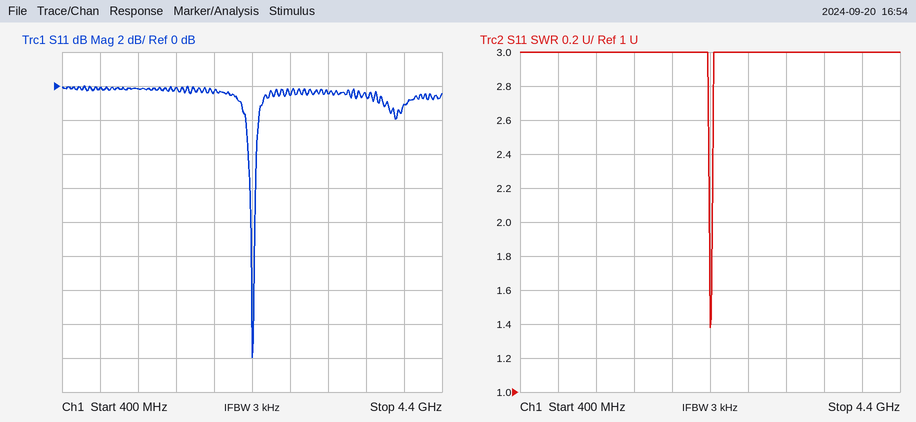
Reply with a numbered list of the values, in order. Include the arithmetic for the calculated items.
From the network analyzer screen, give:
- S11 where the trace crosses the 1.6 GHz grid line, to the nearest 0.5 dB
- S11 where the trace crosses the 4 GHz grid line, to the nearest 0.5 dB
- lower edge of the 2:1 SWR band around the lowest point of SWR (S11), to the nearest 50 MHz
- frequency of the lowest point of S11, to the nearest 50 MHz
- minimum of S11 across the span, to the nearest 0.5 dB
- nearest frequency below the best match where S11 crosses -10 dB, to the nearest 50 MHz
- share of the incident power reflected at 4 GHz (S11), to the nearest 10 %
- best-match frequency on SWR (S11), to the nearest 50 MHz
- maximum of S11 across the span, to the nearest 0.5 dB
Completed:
1. 0.0 dB
2. -1.0 dB
3. 2.40 GHz
4. 2.40 GHz
5. -16.0 dB
6. 2.40 GHz
7. 10^(-1/10) ≈ 79.4 %, so 80 % to the nearest 10 %
8. 2.40 GHz
9. 0.0 dB
